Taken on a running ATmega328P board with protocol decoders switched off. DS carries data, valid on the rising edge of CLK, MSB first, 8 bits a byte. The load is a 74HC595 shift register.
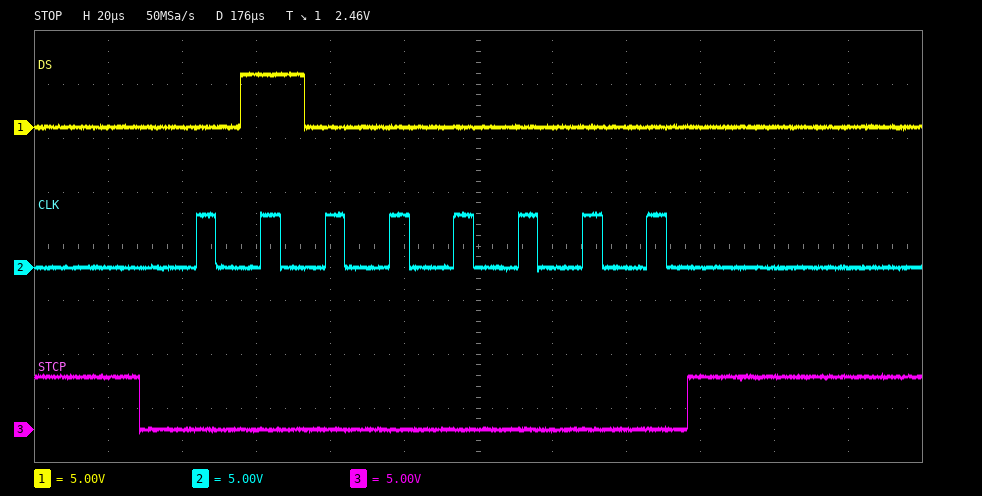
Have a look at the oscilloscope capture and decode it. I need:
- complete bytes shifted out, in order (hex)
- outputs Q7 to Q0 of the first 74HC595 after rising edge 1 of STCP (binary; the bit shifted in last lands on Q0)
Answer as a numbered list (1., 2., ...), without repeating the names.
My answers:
1. 40
2. 01000000
